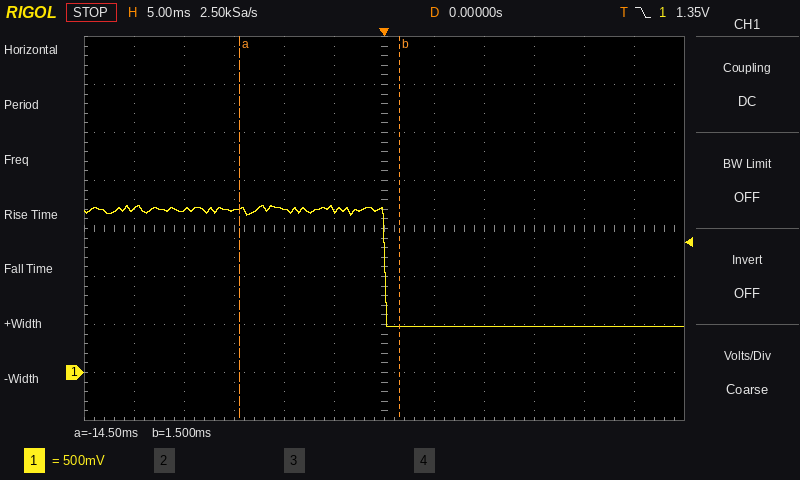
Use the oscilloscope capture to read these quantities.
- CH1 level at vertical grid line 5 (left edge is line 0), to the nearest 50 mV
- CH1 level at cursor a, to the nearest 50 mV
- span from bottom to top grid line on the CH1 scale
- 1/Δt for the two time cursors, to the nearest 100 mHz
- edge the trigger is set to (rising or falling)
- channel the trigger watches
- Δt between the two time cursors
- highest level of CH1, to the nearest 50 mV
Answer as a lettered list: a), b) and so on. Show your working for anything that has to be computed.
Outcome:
a) 1.70 V
b) 1.70 V
c) 4 V
d) 1 / 16.0 ms ≈ 62.5 Hz
e) falling
f) CH1
g) 1.5 ms − (-14.5 ms) = 16.0 ms
h) 1.75 V
